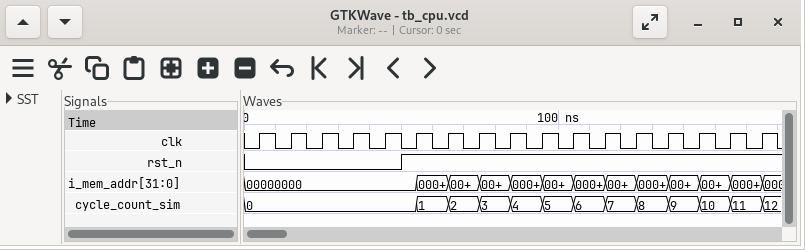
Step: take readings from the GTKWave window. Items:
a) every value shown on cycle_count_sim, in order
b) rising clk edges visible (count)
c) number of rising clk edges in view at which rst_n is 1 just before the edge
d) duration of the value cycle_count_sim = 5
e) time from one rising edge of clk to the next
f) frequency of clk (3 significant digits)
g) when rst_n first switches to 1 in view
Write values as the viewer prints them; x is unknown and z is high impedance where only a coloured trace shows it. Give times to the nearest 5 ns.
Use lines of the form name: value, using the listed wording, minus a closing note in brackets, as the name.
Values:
every value shown on cycle_count_sim, in order: 0, 1, 2, 3, 4, 5, 6, 7, 8, 9, 10, 11, 12
rising clk edges visible: 17
number of rising clk edges in view at which rst_n is 1 just before the edge: 12
duration of the value cycle_count_sim = 5: 10 ns
time from one rising edge of clk to the next: 10 ns
frequency of clk: 100 MHz
when rst_n first switches to 1 in view: 50 ns
